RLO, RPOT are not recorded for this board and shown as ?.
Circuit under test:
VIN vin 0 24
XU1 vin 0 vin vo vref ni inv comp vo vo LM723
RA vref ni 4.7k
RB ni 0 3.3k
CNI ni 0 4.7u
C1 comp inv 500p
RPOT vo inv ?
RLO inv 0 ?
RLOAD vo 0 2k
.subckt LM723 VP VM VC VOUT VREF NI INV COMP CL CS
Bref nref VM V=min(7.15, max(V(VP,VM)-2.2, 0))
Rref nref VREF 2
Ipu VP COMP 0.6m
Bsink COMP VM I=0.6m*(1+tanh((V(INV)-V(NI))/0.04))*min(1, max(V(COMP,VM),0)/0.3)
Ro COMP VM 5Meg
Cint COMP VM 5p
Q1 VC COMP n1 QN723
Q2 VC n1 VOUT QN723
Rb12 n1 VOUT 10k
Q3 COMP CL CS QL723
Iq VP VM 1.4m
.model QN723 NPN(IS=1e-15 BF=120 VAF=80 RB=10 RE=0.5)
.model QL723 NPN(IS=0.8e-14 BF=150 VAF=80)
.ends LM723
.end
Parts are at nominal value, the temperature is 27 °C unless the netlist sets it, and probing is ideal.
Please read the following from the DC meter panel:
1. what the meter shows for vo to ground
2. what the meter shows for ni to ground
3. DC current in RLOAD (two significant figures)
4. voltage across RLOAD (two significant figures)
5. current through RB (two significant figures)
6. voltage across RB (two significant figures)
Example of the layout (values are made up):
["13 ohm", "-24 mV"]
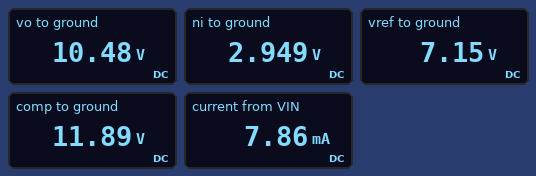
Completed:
["10.48 V", "2.949 V", "5.2 mA", "10 V", "890 µA", "2.9 V"]
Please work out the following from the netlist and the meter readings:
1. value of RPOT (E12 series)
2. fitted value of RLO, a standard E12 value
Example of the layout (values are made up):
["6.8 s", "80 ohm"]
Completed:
["12 kΩ", "4.7 kΩ"]
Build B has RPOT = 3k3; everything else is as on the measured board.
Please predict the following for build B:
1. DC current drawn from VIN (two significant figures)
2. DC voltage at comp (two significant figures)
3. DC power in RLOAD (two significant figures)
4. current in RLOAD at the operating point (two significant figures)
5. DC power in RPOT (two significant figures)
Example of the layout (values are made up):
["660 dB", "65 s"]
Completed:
["5.1 mA", "6.4 V", "13 mW", "2.5 mA", "1.3 mW"]
